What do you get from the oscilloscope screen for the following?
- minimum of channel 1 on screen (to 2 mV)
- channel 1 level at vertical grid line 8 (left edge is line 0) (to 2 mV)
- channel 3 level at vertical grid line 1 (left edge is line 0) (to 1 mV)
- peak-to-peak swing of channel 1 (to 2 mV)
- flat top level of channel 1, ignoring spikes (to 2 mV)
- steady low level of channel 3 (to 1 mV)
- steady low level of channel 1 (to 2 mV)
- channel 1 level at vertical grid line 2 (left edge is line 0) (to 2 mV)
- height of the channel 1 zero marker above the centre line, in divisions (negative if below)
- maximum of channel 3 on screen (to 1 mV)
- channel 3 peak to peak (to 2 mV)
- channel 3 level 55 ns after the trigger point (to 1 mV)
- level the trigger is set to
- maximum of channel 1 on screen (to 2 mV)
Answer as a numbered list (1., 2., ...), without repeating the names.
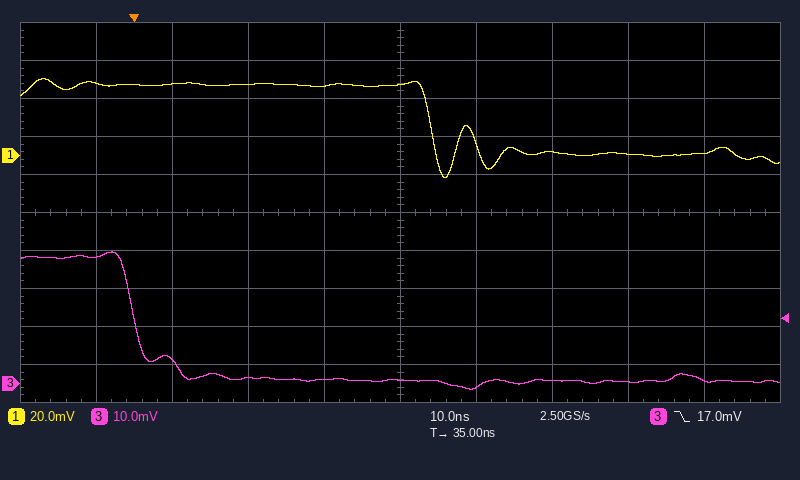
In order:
1. -12 mV
2. 0 mV
3. 33 mV
4. 52 mV
5. 38 mV
6. 1 mV
7. 0 mV
8. 38 mV
9. +1.5 div
10. 35 mV
11. 36 mV
12. 1 mV
13. 17.0 mV
14. 40 mV
